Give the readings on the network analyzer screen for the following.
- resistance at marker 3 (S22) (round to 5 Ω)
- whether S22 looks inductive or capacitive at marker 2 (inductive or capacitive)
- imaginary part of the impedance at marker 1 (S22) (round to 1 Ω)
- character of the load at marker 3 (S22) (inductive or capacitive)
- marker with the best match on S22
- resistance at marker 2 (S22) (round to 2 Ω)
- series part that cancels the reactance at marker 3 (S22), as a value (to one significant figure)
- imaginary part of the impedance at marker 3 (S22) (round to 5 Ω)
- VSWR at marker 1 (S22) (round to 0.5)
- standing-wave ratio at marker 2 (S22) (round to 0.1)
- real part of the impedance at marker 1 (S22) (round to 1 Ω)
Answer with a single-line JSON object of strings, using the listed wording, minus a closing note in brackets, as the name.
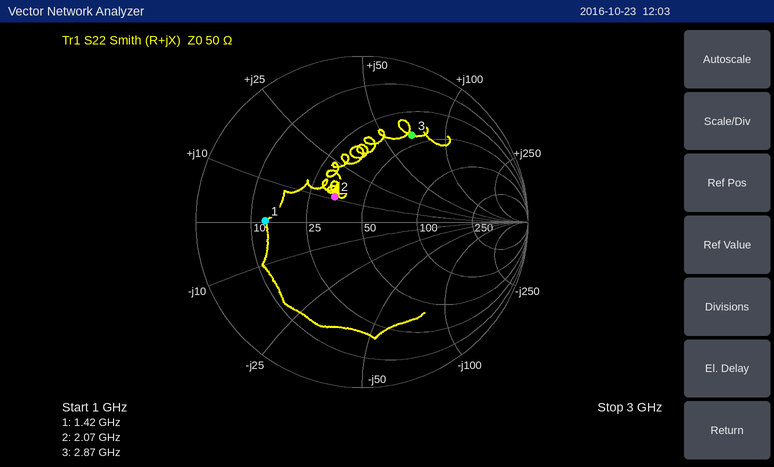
{"resistance at marker 3 (S22)": "40 Ω", "whether S22 looks inductive or capacitive at marker 2": "inductive", "imaginary part of the impedance at marker 1 (S22)": "0 Ω", "character of the load at marker 3 (S22)": "inductive", "marker with the best match on S22": "marker 2", "resistance at marker 2 (S22)": "34 Ω", "series part that cancels the reactance at marker 3 (S22), as a value": "800 fF", "imaginary part of the impedance at marker 3 (S22)": "+70 Ω", "VSWR at marker 1 (S22)": "4.0", "standing-wave ratio at marker 2 (S22)": "1.6", "real part of the impedance at marker 1 (S22)": "13 Ω"}
